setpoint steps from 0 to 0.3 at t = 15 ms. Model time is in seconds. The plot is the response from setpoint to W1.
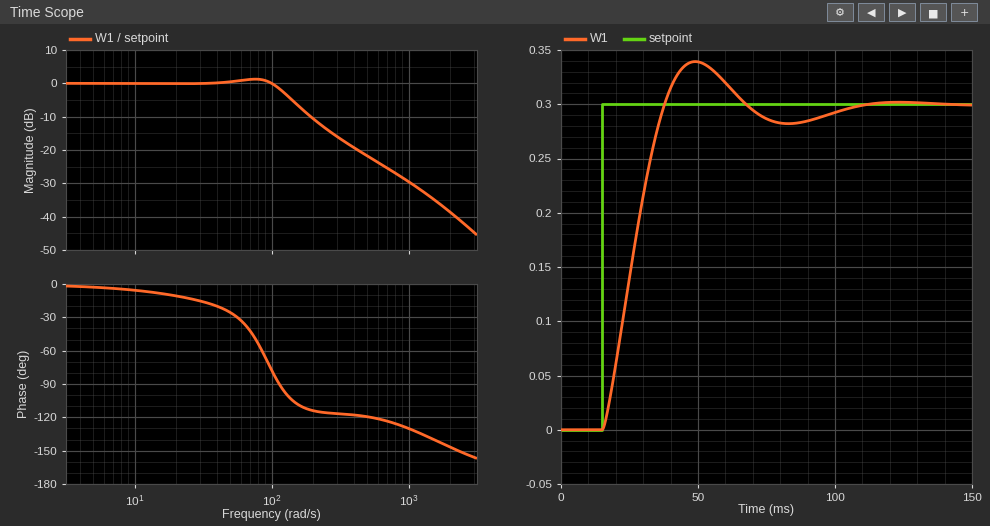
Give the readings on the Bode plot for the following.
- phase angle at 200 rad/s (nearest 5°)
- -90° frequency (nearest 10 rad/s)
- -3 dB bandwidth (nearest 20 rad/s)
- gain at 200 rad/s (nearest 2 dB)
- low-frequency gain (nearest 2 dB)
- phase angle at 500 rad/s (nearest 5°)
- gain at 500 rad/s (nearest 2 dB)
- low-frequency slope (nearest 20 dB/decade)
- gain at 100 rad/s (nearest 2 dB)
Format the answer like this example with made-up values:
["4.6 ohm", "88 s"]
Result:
["-115°", "110 rad/s", "120 rad/s", "-10 dB", "0 dB", "-120°", "-22 dB", "0 dB/decade", "0 dB"]
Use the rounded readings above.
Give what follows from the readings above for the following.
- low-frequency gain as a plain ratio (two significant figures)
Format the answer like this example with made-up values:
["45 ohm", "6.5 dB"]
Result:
["1.0"]
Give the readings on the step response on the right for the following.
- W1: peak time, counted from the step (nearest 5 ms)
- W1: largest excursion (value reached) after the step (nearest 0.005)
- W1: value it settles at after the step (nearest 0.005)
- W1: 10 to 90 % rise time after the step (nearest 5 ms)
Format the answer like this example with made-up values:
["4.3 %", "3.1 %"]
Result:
["35 ms", "0.340", "0.300", "15 ms"]
